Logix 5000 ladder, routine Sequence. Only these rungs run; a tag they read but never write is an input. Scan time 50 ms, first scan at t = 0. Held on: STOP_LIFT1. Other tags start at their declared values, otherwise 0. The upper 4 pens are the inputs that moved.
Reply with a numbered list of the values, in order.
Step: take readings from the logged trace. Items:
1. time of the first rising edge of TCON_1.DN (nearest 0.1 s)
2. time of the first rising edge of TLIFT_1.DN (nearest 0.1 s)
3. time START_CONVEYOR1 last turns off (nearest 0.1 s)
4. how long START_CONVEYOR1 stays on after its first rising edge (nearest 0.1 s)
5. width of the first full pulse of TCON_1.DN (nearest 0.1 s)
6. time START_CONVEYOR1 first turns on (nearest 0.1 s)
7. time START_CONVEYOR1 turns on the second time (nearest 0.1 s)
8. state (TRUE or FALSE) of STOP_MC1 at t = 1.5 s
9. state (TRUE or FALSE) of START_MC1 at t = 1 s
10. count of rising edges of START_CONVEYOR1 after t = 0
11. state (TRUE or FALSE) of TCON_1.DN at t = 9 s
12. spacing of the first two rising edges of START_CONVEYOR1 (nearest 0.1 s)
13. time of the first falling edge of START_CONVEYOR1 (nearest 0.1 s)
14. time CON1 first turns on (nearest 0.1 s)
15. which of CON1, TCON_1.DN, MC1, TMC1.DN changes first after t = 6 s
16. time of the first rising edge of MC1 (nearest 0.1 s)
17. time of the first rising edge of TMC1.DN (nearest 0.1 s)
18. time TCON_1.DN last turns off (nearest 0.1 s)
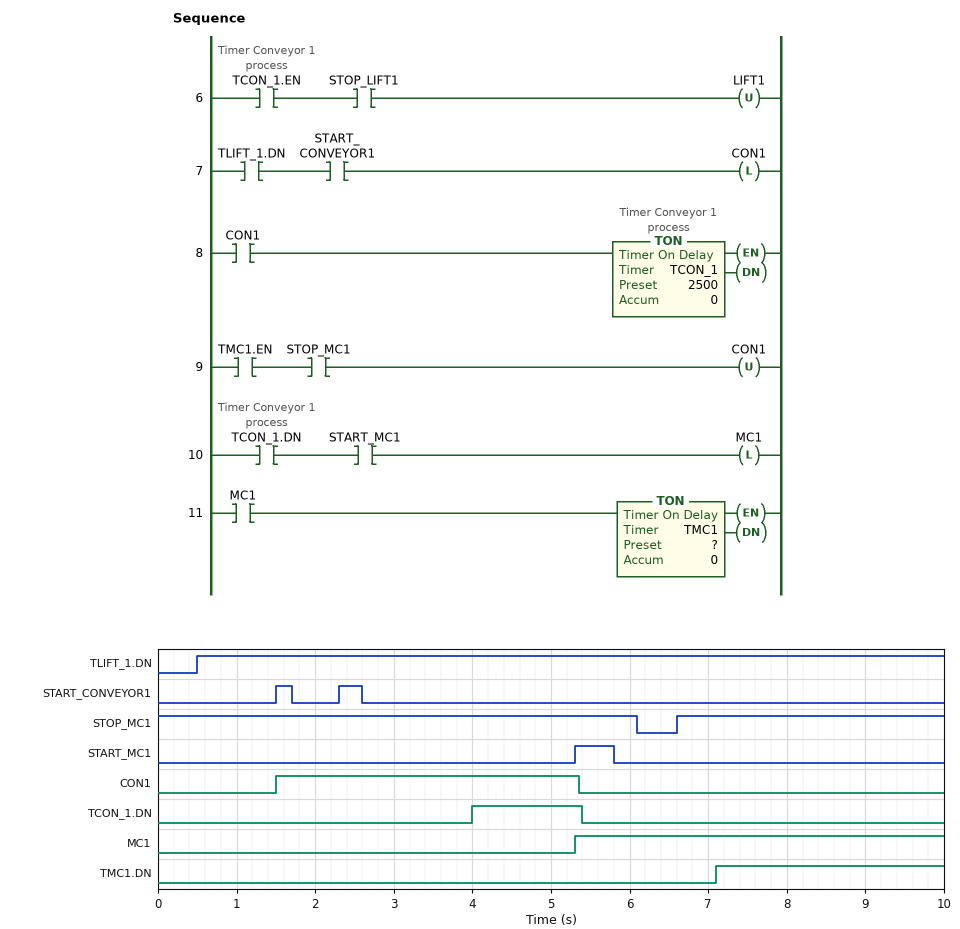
1. 4.0 s
2. 0.5 s
3. 2.6 s
4. 0.2 s
5. 1.4 s
6. 1.5 s
7. 2.3 s
8. TRUE
9. FALSE
10. 2
11. FALSE
12. 0.8 s
13. 1.7 s
14. 1.5 s
15. TMC1.DN
16. 5.3 s
17. 7.1 s
18. 5.4 s
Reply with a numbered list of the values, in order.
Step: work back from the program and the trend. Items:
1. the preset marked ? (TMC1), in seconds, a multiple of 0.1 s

1. 1.8 s
